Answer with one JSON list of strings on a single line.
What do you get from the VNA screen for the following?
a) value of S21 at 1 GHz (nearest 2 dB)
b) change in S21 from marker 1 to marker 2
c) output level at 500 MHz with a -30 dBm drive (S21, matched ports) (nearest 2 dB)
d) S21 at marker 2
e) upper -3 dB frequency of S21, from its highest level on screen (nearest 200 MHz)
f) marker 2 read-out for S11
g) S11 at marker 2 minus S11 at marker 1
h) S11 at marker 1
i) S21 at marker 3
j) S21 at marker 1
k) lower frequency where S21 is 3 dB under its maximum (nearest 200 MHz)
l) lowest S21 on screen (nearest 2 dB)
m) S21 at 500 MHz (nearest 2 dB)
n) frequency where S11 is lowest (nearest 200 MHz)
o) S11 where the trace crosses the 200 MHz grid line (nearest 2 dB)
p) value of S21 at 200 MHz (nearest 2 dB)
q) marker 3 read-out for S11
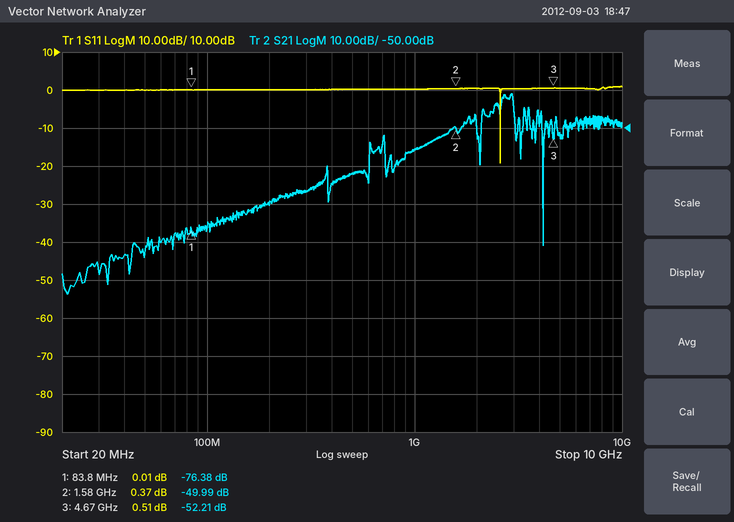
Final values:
["-56 dB", "26.39 dB", "-92 dBm", "-49.99 dB", "3.0 GHz", "0.37 dB", "0.36 dB", "0.01 dB", "-52.21 dB", "-76.38 dB", "2.6 GHz", "-94 dB", "-62 dB", "2.6 GHz", "0 dB", "-70 dB", "0.51 dB"]
